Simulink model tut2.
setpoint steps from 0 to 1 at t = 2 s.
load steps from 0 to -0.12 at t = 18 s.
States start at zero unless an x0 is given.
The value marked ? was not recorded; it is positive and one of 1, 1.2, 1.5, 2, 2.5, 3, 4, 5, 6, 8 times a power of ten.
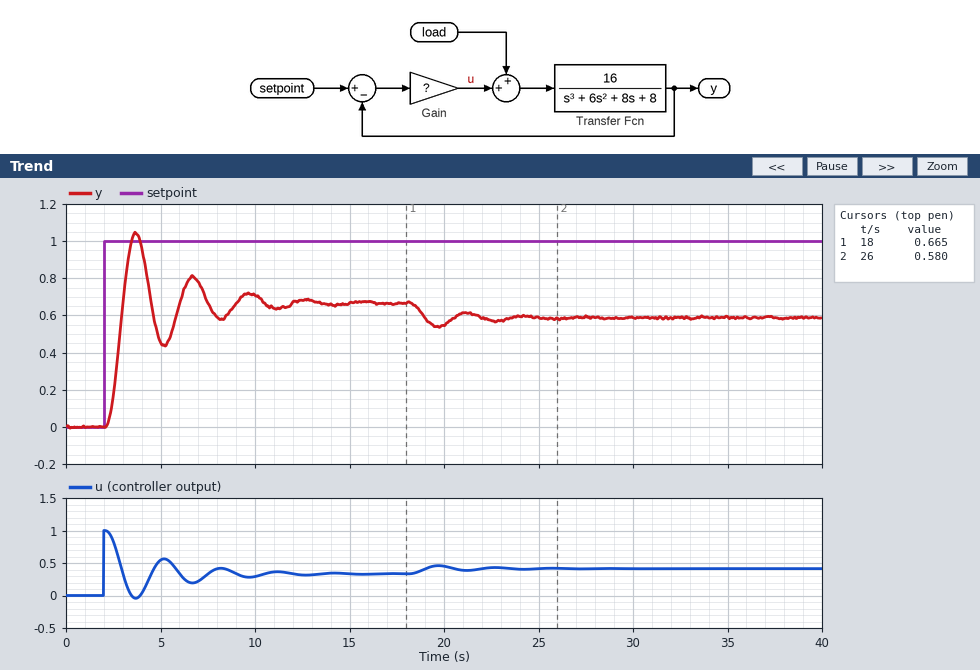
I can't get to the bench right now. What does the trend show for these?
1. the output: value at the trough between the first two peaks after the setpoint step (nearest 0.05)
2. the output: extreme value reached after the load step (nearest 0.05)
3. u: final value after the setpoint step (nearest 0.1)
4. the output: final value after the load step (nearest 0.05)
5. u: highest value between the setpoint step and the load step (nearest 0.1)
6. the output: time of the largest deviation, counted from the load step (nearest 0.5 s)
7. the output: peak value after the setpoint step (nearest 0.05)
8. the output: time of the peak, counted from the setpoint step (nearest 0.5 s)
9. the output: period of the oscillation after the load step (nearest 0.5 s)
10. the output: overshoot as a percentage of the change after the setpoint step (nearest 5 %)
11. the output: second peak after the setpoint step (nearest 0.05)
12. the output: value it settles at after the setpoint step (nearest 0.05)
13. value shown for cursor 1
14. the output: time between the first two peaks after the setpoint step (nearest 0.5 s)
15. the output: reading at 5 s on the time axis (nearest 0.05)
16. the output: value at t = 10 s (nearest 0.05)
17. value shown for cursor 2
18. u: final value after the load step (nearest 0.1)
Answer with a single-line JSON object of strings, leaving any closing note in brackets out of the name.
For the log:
{"the output: value at the trough between the first two peaks after the setpoint step": "0.45", "the output: extreme value reached after the load step": "0.55", "u: final value after the setpoint step": "0.3", "the output: final value after the load step": "0.60", "u: highest value between the setpoint step and the load step": "1.0", "the output: time of the largest deviation, counted from the load step": "1.5 s", "the output: peak value after the setpoint step": "1.05", "the output: time of the peak, counted from the setpoint step": "1.5 s", "the output: period of the oscillation after the load step": "3.0 s", "the output: overshoot as a percentage of the change after the setpoint step": "55 %", "the output: second peak after the setpoint step": "0.80", "the output: value it settles at after the setpoint step": "0.65", "value shown for cursor 1": "0.665", "the output: time between the first two peaks after the setpoint step": "3.0 s", "the output: reading at 5 s on the time axis": "0.45", "the output: value at t = 10 s": "0.70", "value shown for cursor 2": "0.580", "u: final value after the load step": "0.4"}
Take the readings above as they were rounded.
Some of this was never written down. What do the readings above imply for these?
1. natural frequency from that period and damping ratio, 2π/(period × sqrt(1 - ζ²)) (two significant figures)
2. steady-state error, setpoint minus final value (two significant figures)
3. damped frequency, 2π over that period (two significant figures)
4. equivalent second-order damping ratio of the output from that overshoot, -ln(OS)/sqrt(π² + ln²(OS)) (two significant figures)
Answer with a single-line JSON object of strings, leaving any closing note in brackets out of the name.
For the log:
{"natural frequency from that period and damping ratio, 2π/(period × sqrt(1 - ζ²))": "2.1 rad/s", "steady-state error, setpoint minus final value": "0.35", "damped frequency, 2π over that period": "2.1 rad/s", "equivalent second-order damping ratio of the output from that overshoot, -ln(OS)/sqrt(π² + ln²(OS))": "0.19"}
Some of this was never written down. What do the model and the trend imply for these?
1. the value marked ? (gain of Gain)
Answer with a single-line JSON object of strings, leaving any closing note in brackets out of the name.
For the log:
{"the value marked ?": "1"}
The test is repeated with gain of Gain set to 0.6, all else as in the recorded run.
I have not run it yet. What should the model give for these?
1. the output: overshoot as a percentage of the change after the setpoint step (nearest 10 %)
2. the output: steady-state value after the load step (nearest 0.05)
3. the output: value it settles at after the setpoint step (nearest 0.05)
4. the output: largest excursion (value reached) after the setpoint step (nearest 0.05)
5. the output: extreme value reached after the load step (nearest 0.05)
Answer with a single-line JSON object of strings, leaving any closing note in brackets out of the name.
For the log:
{"the output: overshoot as a percentage of the change after the setpoint step": "40 %", "the output: steady-state value after the load step": "0.45", "the output: value it settles at after the setpoint step": "0.55", "the output: largest excursion (value reached) after the setpoint step": "0.80", "the output: extreme value reached after the load step": "0.40"}
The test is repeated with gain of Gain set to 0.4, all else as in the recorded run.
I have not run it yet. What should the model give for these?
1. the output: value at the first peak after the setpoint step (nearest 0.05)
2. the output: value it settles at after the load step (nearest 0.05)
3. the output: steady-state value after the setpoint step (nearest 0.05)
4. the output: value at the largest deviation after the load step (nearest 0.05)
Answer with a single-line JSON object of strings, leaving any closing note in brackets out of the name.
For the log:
{"the output: value at the first peak after the setpoint step": "0.60", "the output: value it settles at after the load step": "0.30", "the output: steady-state value after the setpoint step": "0.45", "the output: value at the largest deviation after the load step": "0.25"}
